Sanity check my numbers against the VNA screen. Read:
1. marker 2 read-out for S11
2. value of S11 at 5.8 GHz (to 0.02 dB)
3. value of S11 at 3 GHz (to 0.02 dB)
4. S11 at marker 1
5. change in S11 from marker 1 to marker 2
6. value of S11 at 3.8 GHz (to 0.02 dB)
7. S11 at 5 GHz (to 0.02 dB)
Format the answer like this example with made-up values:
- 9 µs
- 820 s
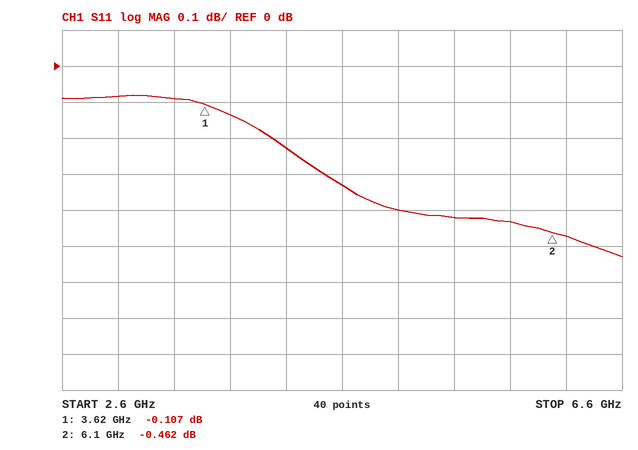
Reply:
- -0.462 dB
- -0.44 dB
- -0.08 dB
- -0.107 dB
- -0.355 dB
- -0.14 dB
- -0.40 dB
